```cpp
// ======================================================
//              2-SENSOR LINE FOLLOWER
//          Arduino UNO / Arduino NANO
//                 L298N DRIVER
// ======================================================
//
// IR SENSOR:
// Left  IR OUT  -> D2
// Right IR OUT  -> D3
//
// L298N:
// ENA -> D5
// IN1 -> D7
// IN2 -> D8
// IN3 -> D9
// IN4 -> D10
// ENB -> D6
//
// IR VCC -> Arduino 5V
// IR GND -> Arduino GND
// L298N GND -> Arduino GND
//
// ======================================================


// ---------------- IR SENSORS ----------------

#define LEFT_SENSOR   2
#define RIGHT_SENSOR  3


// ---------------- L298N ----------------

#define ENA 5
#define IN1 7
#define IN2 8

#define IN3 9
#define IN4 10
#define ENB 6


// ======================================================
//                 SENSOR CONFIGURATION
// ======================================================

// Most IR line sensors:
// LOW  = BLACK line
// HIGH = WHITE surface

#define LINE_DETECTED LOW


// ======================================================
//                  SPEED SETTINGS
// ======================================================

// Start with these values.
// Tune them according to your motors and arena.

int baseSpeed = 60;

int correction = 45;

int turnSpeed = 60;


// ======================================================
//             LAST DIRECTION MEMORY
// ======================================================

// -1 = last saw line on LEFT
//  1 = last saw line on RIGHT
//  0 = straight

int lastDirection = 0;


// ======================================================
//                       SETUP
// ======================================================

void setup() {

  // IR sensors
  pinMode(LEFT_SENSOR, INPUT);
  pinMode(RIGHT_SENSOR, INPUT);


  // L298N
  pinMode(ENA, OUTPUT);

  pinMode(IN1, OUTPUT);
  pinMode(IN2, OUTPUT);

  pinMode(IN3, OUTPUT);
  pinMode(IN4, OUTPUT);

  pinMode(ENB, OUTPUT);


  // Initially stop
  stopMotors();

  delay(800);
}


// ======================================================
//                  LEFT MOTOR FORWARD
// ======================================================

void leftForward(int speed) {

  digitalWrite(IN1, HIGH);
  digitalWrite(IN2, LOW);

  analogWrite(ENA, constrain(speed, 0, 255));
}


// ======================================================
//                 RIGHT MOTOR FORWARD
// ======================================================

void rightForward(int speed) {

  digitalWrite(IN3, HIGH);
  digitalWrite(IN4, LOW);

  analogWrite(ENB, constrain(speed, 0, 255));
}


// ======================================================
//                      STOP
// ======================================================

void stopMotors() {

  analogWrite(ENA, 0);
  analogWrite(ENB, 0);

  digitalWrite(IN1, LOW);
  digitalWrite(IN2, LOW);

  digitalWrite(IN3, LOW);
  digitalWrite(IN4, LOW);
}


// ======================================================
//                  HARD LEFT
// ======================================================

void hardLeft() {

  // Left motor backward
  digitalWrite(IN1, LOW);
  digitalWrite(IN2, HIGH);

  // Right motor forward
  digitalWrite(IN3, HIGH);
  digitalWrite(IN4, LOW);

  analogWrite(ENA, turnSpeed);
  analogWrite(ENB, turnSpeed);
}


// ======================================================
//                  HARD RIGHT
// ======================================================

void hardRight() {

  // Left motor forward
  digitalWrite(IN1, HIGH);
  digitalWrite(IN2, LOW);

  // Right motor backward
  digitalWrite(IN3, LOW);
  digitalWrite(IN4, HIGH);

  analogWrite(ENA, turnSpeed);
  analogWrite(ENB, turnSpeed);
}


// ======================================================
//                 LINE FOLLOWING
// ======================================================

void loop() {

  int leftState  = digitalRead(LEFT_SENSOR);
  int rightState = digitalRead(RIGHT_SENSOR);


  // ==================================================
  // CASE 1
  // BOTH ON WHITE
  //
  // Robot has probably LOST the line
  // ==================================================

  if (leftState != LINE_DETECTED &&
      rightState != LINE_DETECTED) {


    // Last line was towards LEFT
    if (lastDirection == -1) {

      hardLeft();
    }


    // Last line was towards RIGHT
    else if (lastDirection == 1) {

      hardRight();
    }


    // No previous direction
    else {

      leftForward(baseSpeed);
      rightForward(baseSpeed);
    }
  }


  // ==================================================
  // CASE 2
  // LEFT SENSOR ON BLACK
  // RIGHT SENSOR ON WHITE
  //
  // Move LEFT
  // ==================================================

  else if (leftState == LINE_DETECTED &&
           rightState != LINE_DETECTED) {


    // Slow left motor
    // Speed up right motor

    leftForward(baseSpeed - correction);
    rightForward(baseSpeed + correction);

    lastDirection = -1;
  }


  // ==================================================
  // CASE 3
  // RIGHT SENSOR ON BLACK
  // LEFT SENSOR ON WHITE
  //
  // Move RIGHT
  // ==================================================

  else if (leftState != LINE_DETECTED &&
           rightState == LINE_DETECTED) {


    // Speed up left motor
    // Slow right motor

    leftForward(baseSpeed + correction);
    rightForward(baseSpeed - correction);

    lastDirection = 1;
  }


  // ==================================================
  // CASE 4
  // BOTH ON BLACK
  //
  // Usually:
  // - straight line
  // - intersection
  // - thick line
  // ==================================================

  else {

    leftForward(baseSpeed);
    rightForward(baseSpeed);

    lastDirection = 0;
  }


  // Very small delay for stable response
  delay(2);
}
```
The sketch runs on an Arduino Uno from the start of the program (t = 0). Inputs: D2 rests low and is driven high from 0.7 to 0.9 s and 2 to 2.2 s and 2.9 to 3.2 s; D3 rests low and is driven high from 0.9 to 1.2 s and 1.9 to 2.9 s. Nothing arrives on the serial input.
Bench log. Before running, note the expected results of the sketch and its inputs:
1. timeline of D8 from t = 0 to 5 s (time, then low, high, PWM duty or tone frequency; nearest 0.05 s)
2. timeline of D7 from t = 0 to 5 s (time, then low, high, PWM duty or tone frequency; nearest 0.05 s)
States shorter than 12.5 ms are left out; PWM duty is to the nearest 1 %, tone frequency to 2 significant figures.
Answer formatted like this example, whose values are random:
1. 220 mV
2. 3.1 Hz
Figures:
1. 0 s low; 2 s high; 2.2 s low
2. 0 s low; 0.8 s high; 2 s low; 2.2 s high
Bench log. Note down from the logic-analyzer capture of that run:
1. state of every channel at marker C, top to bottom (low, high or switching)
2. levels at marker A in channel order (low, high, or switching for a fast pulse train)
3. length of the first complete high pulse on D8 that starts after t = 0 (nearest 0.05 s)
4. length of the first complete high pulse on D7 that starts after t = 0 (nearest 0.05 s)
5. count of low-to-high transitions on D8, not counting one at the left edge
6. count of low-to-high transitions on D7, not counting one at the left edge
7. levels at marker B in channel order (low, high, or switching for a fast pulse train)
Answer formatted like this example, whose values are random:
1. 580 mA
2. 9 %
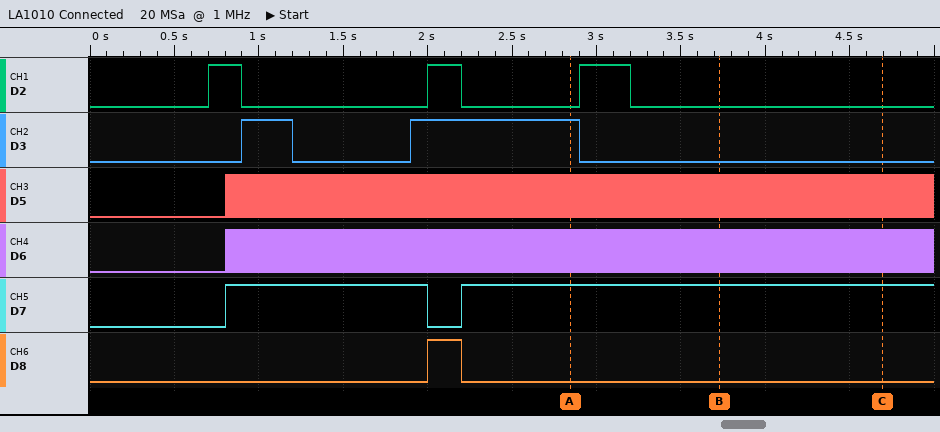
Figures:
1. D2 low, D3 low, D5 switching, D6 switching, D7 high, D8 low
2. D2 low, D3 high, D5 switching, D6 switching, D7 high, D8 low
3. 0.20 s
4. 1.20 s
5. 1
6. 2
7. D2 low, D3 low, D5 switching, D6 switching, D7 high, D8 low
